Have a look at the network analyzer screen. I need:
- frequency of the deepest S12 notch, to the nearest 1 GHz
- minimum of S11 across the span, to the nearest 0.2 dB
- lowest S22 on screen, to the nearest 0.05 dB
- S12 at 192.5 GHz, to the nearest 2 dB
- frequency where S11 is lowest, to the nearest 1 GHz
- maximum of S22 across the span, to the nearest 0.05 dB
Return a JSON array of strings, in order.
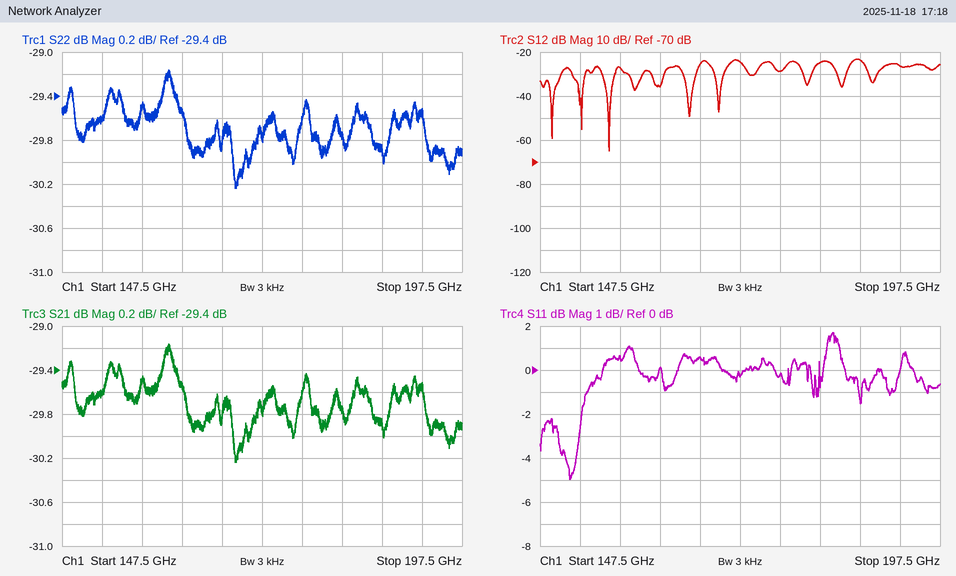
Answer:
["156 GHz", "-5.0 dB", "-30.25 dB", "-26 dB", "151 GHz", "-29.15 dB"]
